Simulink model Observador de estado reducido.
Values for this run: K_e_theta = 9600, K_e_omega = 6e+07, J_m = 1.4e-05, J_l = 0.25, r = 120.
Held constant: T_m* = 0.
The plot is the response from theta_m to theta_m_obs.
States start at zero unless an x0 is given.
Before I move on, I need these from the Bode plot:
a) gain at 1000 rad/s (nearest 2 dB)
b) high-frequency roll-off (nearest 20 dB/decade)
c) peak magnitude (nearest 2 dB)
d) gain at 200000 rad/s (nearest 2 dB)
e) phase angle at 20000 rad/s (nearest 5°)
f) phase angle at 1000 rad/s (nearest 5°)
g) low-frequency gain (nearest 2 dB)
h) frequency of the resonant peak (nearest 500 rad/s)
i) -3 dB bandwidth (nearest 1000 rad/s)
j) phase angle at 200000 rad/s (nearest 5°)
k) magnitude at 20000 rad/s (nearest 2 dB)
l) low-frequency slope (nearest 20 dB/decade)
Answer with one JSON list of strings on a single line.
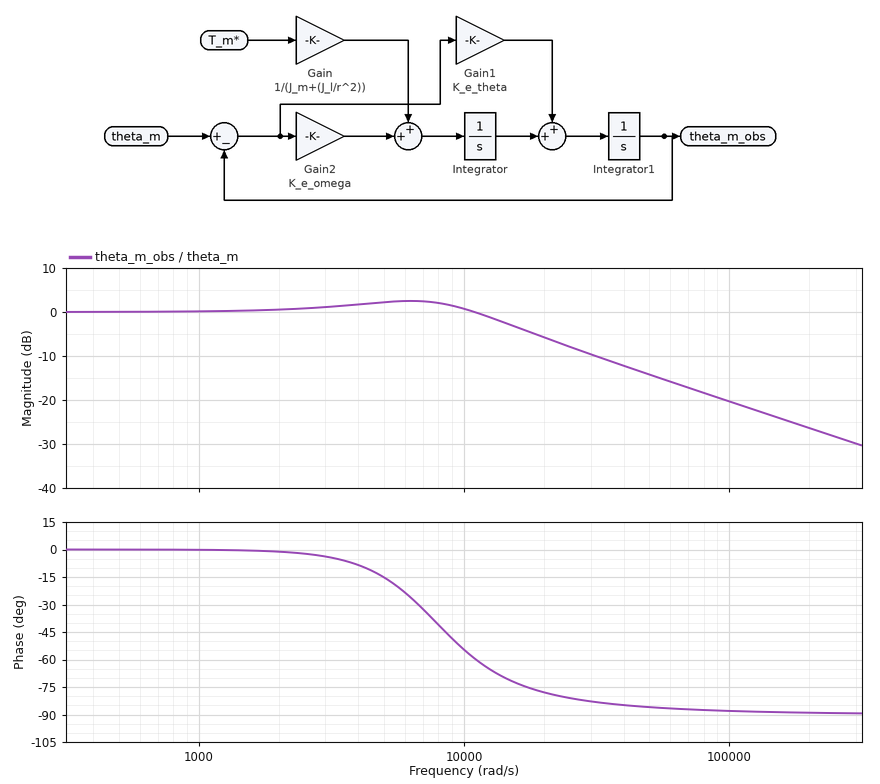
["0 dB", "-20 dB/decade", "2 dB", "-26 dB", "-80°", "0°", "0 dB", "6000 rad/s", "15000 rad/s", "-90°", "-6 dB", "0 dB/decade"]
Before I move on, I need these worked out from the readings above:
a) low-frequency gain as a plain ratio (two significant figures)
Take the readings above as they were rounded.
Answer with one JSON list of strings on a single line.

["1.0"]
